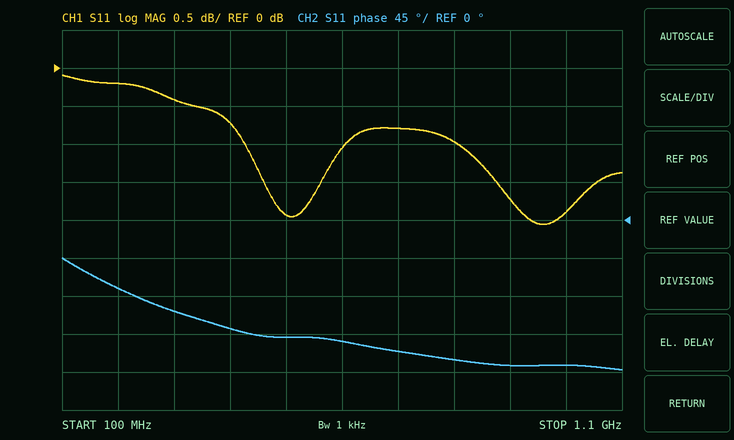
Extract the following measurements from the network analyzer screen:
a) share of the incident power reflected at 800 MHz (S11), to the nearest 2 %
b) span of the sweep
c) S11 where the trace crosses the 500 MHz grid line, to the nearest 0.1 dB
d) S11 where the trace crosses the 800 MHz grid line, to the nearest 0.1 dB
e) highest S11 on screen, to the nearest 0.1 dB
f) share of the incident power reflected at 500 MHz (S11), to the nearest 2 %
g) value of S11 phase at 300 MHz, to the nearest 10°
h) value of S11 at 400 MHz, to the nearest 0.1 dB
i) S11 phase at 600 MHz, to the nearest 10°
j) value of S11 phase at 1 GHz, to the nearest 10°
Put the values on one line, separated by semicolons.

80 %; 1 GHz; -1.9 dB; -1.0 dB; -0.1 dB; 64 %; -110°; -0.7 dB; -140°; -170°
